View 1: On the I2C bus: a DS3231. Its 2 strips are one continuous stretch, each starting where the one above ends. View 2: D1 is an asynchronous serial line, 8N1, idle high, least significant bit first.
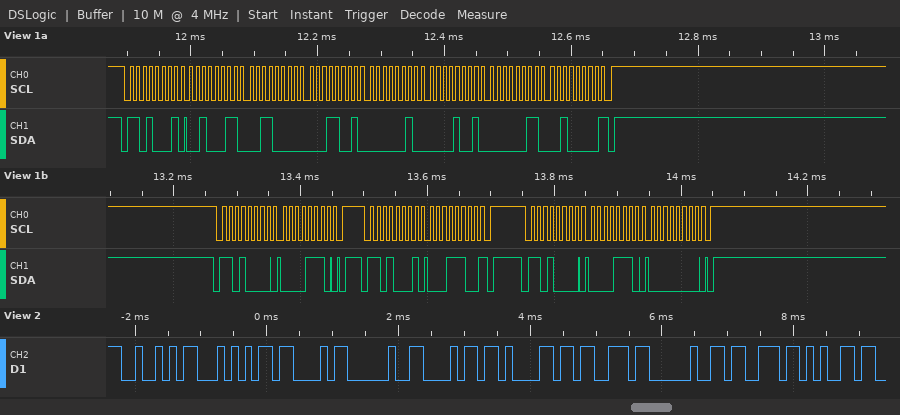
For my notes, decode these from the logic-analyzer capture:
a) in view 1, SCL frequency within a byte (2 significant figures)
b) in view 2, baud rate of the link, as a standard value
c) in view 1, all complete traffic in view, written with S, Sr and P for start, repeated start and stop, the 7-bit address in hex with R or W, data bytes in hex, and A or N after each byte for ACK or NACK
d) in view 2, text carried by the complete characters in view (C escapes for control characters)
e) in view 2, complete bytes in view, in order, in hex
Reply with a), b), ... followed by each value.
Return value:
a) 100 kHz
b) 9600 baud
c) S 68R A 23 A 30 A 19 A 02 A 09 A 03 A 20 N P S 68W A 0E A P S 68R A 1C N P S 68W A 0E A 00 A P
d) "RTC has se"
e) 52 54 43 20 68 61 73 20 73 65
